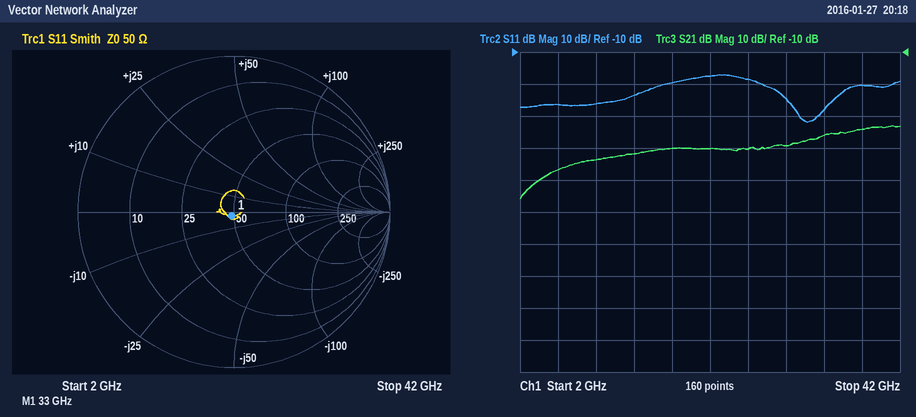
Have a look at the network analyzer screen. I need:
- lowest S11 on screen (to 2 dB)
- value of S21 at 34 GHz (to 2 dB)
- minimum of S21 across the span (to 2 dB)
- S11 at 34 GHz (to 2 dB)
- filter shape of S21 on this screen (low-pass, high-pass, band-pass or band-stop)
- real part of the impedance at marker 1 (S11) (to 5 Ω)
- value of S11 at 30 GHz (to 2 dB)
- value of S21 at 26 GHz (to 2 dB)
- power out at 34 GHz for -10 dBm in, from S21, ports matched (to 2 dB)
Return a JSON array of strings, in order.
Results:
["-32 dB", "-36 dB", "-56 dB", "-28 dB", "high-pass", "50 Ω", "-24 dB", "-40 dB", "-46 dBm"]
